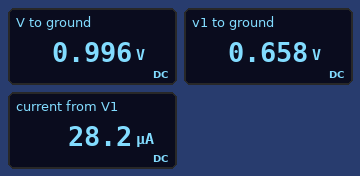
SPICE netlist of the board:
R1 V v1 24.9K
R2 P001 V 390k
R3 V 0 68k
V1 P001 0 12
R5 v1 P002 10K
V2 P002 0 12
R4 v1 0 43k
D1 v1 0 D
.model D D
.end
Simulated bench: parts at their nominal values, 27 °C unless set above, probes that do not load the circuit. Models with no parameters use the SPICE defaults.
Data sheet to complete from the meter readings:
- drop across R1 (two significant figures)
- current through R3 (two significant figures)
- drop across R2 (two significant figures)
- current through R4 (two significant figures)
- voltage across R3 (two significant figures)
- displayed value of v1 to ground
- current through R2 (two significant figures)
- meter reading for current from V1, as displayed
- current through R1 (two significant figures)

340 mV
15 µA
11 V
15 µA
1.0 V
0.658 V
28 µA
28.2 µA
14 µA
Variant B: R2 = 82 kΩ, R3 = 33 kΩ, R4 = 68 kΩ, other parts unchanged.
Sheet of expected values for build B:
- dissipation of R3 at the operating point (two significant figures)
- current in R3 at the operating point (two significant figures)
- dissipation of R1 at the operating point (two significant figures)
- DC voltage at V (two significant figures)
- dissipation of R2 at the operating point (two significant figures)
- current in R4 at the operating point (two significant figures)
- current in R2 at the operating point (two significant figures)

130 µW
63 µA
82 µW
2.1 V
1.2 mW
9.7 µA
120 µA
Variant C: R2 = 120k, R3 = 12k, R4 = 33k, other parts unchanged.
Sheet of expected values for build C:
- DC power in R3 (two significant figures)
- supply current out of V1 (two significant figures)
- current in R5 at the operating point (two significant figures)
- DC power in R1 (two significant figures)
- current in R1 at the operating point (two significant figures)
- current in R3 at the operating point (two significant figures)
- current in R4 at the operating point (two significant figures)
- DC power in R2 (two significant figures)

77 µW
92 µA
1.1 mA
3.6 µW
12 µA
80 µA
20 µA
1.0 mW
